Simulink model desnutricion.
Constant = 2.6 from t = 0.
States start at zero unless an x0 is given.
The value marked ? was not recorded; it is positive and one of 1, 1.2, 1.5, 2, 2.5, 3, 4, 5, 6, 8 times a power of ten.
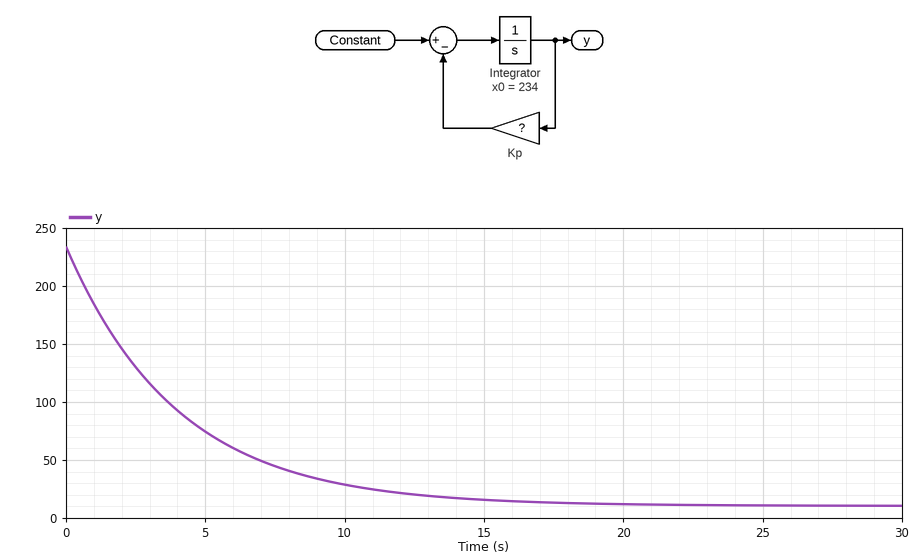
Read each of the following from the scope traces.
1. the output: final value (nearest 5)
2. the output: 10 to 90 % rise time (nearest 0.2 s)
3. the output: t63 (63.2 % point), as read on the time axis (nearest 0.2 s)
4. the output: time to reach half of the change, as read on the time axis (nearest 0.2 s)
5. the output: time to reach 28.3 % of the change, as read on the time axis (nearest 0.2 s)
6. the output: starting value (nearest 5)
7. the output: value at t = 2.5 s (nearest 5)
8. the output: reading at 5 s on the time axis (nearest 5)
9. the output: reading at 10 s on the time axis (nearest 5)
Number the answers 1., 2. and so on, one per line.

1. 10
2. 8.8 s
3. 4.0 s
4. 2.8 s
5. 1.4 s
6. 235
7. 130
8. 75
9. 30
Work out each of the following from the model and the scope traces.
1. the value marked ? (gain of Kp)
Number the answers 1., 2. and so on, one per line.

1. 0.25
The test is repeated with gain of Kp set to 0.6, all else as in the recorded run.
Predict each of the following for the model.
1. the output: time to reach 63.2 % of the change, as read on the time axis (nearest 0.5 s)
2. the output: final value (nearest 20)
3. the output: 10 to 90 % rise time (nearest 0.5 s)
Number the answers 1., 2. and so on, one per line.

1. 1.5 s
2. 0
3. 3.5 s
